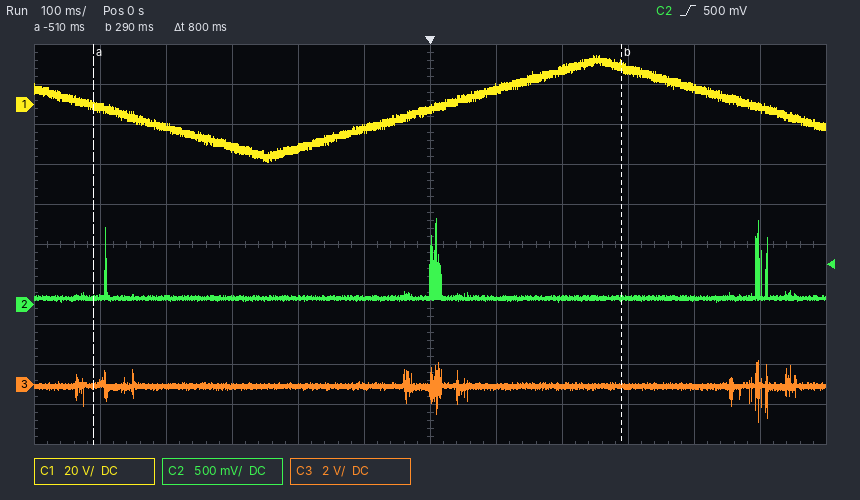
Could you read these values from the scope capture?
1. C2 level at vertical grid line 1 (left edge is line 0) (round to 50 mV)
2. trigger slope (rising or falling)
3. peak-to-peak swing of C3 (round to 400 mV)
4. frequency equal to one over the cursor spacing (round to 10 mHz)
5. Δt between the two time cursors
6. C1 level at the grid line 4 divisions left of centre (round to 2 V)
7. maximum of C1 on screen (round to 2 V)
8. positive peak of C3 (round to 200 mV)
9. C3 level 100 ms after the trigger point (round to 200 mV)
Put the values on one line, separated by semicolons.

100 mV; rising; 3.2 V; 1.25 Hz; 800 ms; -12 V; 24 V; 1.2 V; -200 mV
